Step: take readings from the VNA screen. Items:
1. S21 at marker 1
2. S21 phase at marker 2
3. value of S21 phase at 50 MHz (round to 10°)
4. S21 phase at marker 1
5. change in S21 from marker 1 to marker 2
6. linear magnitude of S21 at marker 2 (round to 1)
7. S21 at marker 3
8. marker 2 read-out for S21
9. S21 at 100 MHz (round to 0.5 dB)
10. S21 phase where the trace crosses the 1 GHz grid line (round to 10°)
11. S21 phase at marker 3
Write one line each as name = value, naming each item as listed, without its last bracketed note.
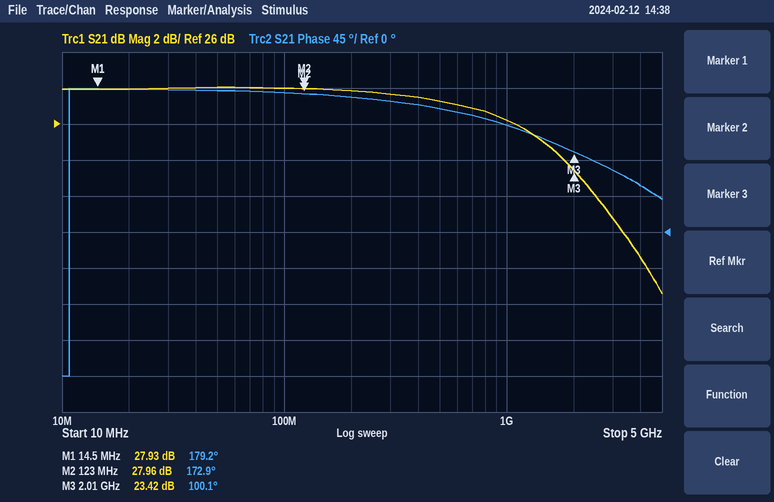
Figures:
S21 at marker 1 = 27.93 dB
S21 phase at marker 2 = 172.9°
value of S21 phase at 50 MHz = 180°
S21 phase at marker 1 = 179.2°
change in S21 from marker 1 to marker 2 = 0.03 dB
linear magnitude of S21 at marker 2 = 25
S21 at marker 3 = 23.42 dB
marker 2 read-out for S21 = 27.96 dB
S21 at 100 MHz = 28.0 dB
S21 phase where the trace crosses the 1 GHz grid line = 130°
S21 phase at marker 3 = 100.1°
